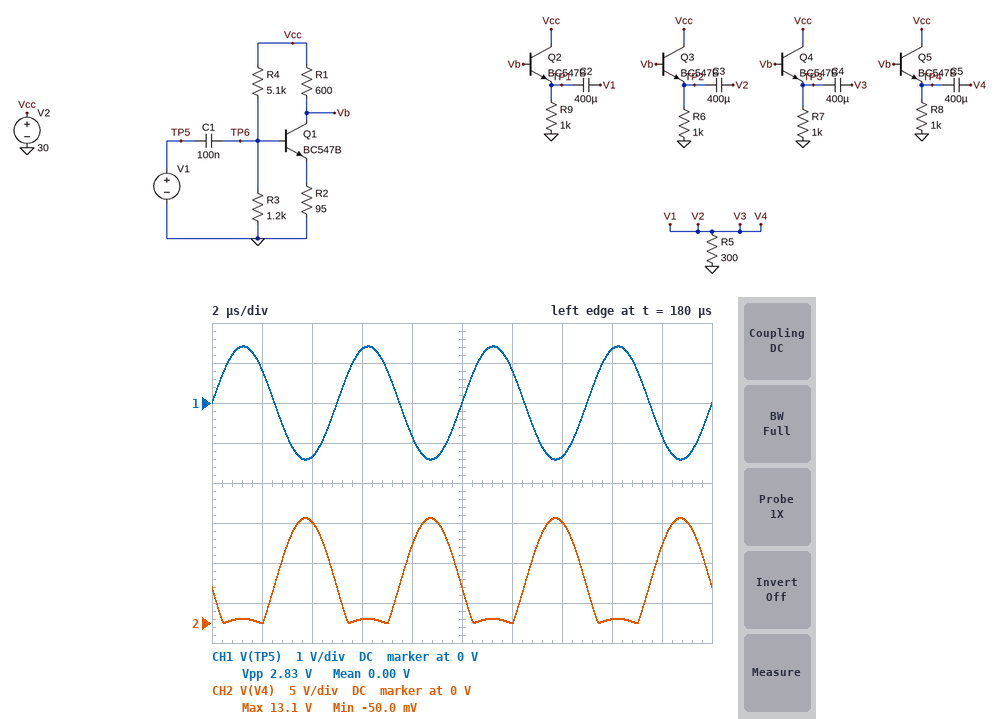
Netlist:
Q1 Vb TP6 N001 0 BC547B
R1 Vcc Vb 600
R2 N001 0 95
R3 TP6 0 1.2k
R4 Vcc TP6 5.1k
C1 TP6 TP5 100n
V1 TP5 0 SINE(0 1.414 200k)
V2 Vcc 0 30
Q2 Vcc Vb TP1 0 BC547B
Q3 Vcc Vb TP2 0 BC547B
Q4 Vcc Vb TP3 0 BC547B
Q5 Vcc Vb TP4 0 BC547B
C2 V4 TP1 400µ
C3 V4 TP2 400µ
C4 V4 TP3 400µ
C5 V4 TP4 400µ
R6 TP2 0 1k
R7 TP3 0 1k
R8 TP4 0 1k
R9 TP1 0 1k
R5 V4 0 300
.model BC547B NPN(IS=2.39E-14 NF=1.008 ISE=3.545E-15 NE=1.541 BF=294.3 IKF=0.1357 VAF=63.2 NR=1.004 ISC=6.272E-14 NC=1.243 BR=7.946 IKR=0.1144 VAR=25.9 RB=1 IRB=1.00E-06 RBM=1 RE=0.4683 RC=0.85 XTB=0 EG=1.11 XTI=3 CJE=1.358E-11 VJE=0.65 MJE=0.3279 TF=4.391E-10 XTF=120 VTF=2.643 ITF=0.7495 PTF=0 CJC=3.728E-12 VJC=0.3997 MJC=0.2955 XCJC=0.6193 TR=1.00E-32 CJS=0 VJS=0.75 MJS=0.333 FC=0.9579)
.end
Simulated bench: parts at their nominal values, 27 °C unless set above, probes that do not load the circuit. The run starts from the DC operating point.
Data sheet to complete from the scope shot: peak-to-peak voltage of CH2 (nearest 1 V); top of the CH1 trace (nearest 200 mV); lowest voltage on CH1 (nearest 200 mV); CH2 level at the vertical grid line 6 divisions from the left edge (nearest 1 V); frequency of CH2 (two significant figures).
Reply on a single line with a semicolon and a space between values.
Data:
13 V; 1.4 V; -1.4 V; 0 V; 200 kHz
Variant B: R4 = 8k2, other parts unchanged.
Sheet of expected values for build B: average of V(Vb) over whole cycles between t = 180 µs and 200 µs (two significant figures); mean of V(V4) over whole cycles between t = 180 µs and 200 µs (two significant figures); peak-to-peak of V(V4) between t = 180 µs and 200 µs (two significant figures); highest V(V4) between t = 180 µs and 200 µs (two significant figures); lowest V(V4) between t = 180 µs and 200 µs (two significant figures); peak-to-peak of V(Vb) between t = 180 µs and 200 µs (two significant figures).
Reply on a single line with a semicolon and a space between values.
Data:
12 V; 1.1 V; 15 V; 9.3 V; -5.8 V; 16 V
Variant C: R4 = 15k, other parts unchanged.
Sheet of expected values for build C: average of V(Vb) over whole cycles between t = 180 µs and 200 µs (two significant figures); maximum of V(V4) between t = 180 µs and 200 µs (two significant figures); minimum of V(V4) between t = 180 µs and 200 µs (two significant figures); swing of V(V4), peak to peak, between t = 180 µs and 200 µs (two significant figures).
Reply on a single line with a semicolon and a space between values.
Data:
21 V; 8.2 V; -8.5 V; 17 V
